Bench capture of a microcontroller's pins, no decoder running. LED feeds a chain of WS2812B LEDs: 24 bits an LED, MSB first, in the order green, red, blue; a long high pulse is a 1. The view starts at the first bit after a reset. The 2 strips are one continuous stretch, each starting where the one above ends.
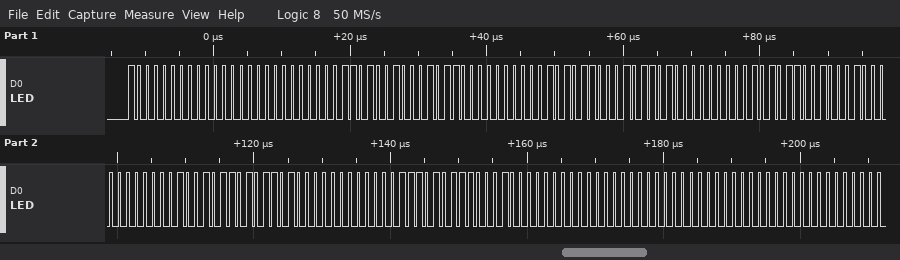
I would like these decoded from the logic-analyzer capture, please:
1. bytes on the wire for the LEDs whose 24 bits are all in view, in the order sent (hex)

80 00 00 69 16 00 56 2D 00 56 44 00 4B 5A 00 1D 71 00 00 00 00
